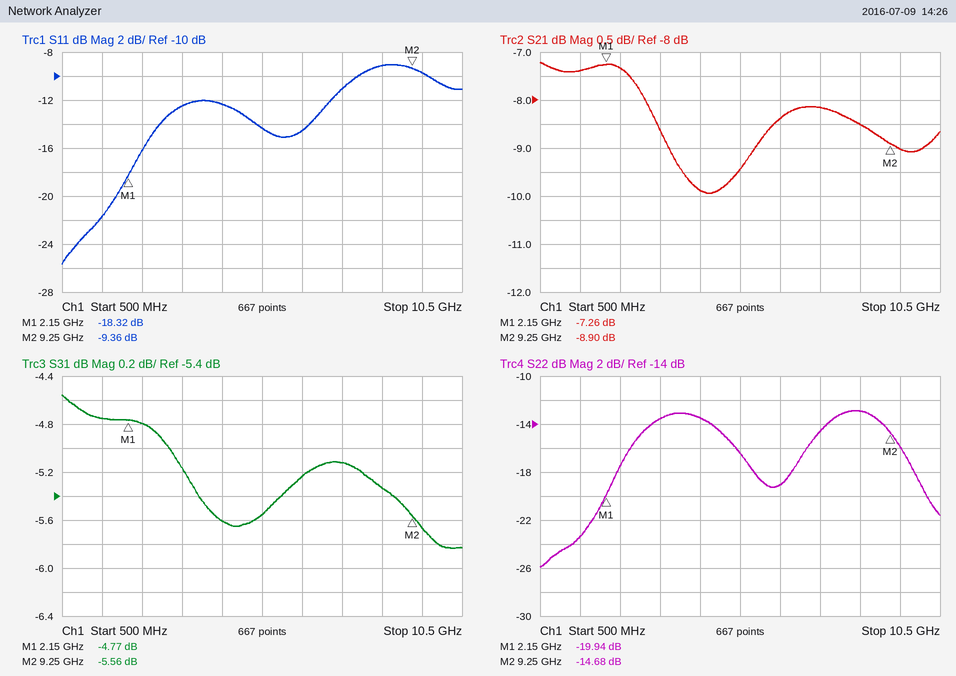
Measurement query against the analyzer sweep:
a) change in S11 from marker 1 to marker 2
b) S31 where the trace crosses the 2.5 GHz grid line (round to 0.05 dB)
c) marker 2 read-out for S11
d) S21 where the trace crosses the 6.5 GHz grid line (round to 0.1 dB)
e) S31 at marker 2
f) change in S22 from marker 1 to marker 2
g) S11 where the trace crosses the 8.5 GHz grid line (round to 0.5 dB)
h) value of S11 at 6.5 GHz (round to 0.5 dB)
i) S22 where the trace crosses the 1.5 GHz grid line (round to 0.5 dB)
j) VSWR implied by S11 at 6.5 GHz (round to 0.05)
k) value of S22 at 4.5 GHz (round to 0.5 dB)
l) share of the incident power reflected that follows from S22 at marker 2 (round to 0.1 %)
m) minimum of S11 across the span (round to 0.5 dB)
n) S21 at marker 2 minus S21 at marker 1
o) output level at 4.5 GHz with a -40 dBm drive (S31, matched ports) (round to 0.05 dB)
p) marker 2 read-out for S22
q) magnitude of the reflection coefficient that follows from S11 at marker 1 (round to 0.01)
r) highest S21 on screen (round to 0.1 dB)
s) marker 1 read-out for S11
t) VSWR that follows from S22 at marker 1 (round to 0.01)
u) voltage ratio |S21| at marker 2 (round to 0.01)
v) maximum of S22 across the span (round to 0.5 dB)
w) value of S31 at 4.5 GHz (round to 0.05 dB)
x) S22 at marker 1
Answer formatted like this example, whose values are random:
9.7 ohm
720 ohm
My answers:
8.96 dB
-4.80 dB
-9.36 dB
-8.4 dB
-5.56 dB
5.26 dB
-9.0 dB
-14.5 dB
-23.5 dB
1.45
-13.5 dB
3.4 %
-25.5 dB
-1.64 dB
-45.60 dBm
-14.68 dB
0.12
-7.2 dB
-18.32 dB
1.22
0.36
-13.0 dB
-5.60 dB
-19.94 dB
